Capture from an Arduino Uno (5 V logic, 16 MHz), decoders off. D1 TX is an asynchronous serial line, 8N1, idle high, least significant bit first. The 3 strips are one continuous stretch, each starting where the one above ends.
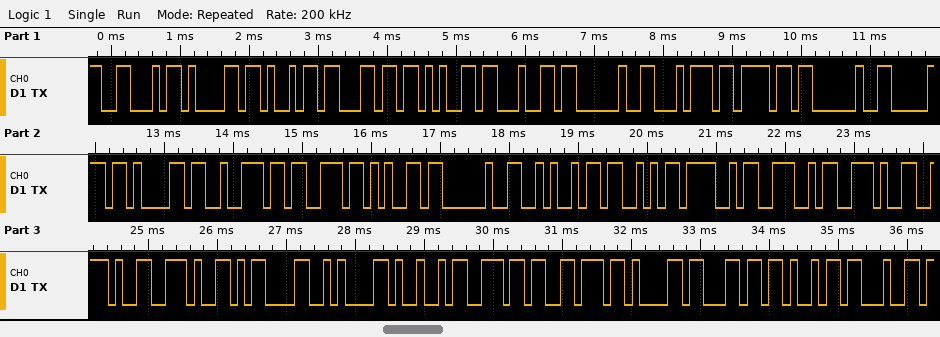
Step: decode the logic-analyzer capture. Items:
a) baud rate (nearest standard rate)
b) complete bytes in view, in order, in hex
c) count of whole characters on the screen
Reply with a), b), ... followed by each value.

a) 9600 baud
b) 46 61 69 6C 65 64 20 74 6F 20 70 61 72 73 65 20 4A 53 4F 4E 2E 2E 2E 0D 0A 49 6E 76 61 6C 69 64
c) 32
